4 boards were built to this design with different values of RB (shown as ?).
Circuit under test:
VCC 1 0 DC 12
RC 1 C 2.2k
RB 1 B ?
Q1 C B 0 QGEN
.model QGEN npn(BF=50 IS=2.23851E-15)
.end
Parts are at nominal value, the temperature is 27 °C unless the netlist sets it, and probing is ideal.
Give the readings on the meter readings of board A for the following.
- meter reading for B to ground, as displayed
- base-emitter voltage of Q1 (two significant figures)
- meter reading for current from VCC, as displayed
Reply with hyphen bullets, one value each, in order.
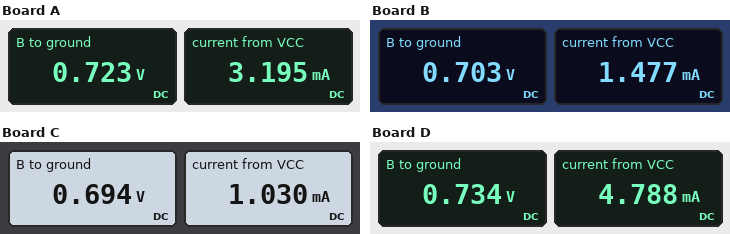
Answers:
- 0.723 V
- 720 mV
- 3.195 mA
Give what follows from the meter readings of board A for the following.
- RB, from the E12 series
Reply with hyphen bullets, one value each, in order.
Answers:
- 180 kΩ
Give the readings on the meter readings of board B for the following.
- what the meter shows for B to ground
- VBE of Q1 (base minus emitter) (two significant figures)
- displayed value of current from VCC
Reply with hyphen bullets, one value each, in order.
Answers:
- 0.703 V
- 700 mV
- 1.477 mA
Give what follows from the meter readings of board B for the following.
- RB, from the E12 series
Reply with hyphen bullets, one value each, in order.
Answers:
- 390 kΩ
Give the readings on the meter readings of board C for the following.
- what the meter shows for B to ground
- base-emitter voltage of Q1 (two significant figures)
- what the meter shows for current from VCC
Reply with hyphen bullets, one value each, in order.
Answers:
- 0.694 V
- 690 mV
- 1.030 mA
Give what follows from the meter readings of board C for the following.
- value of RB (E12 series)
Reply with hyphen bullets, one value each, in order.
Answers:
- 560 kΩ
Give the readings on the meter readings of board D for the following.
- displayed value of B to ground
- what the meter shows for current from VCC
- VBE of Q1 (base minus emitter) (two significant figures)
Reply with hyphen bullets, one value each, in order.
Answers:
- 0.734 V
- 4.788 mA
- 730 mV
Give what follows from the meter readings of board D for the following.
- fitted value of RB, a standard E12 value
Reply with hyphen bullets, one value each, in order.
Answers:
- 120 kΩ
